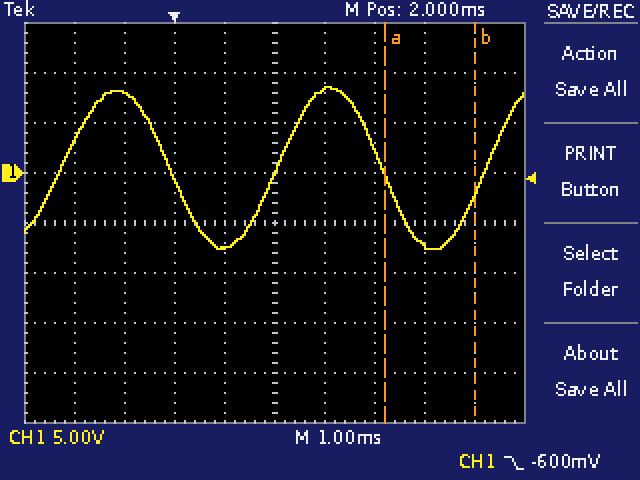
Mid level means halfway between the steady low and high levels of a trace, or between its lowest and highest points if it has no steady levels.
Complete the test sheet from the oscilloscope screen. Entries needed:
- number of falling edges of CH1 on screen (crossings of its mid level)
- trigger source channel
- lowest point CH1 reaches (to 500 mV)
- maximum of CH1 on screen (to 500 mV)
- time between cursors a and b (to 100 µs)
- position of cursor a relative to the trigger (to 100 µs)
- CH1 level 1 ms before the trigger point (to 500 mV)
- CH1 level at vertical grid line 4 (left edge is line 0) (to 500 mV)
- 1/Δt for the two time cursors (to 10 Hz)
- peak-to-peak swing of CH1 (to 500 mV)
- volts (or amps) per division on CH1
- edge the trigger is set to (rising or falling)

2
CH1
-7.5 V
8.5 V
1.8 ms
+4.2 ms
8.0 V
-7.5 V
560 Hz
16.0 V
5 V
falling
